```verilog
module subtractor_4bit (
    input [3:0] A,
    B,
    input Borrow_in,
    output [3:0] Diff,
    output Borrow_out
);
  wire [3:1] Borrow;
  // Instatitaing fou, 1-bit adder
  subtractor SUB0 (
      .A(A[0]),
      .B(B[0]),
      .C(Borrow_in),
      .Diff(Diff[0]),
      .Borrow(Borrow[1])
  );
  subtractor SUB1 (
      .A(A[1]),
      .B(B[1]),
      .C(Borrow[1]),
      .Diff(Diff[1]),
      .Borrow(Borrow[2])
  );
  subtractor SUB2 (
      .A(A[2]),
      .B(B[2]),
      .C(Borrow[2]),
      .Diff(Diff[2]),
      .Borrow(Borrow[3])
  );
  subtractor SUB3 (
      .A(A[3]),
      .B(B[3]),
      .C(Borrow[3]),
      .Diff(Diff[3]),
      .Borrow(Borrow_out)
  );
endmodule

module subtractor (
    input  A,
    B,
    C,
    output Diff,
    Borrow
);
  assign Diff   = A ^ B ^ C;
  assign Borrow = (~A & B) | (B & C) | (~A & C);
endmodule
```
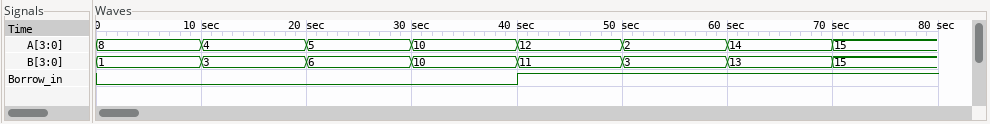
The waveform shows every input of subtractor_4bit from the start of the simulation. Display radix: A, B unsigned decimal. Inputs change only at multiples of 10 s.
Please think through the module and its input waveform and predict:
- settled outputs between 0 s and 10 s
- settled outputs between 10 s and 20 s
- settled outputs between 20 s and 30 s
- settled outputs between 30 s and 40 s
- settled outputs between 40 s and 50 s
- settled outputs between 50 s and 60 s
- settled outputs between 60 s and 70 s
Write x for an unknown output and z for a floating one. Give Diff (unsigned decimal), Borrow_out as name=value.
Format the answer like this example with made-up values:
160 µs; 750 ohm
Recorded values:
Diff=7, Borrow_out=0; Diff=1, Borrow_out=0; Diff=15, Borrow_out=1; Diff=0, Borrow_out=0; Diff=0, Borrow_out=0; Diff=14, Borrow_out=1; Diff=0, Borrow_out=0
